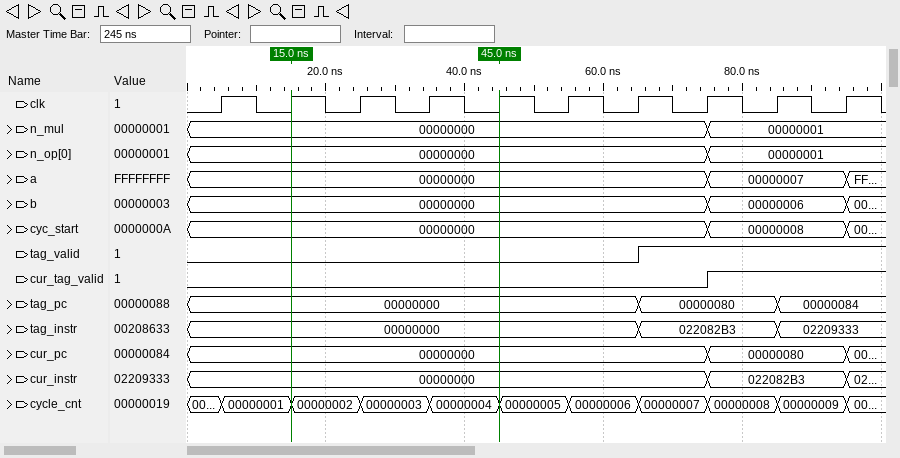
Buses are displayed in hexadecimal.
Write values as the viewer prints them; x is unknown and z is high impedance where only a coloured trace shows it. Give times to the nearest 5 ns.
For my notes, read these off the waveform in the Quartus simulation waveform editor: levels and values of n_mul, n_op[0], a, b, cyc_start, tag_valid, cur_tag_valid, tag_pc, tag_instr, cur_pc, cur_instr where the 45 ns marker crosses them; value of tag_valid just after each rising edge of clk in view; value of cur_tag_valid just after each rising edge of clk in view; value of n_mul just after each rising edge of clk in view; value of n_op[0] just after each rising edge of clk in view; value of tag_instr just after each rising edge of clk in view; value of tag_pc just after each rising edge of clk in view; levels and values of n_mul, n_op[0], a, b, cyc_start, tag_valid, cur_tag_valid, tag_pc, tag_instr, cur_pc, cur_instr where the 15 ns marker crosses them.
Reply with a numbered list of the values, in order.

1. n_mul=00000000, n_op[0]=00000000, a=00000000, b=00000000, cyc_start=00000000, tag_valid=0, cur_tag_valid=0, tag_pc=00000000, tag_instr=00000000, cur_pc=00000000, cur_instr=00000000
2. 0 0 0 0 0 0 1 1 1 1
3. 0 0 0 0 0 0 0 1 1 1
4. 00000000, 00000000, 00000000, 00000000, 00000000, 00000000, 00000000, 00000001, 00000001, 00000001
5. 00000000, 00000000, 00000000, 00000000, 00000000, 00000000, 00000000, 00000001, 00000001, 00000001
6. 00000000, 00000000, 00000000, 00000000, 00000000, 00000000, 022082B3, 022082B3, 02209333, 02209333
7. 00000000, 00000000, 00000000, 00000000, 00000000, 00000000, 00000080, 00000080, 00000084, 00000084
8. n_mul=00000000, n_op[0]=00000000, a=00000000, b=00000000, cyc_start=00000000, tag_valid=0, cur_tag_valid=0, tag_pc=00000000, tag_instr=00000000, cur_pc=00000000, cur_instr=00000000
